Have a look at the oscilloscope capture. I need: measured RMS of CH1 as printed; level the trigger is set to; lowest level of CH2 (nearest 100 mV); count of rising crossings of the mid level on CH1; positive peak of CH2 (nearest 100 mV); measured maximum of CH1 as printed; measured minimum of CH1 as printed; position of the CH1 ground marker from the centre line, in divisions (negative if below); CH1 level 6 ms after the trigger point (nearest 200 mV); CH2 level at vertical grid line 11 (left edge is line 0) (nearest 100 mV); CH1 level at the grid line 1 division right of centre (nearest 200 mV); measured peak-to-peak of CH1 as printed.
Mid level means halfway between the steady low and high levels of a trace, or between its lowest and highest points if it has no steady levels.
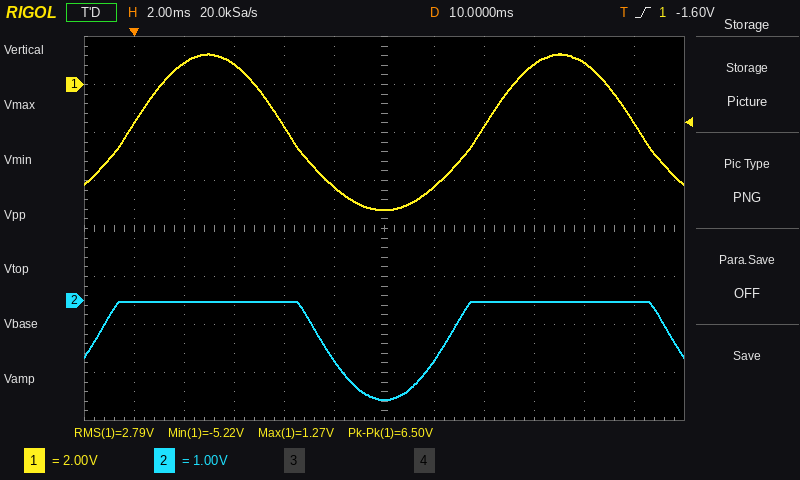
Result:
2.79 V
-1.60 V
-2.1 V
2
0.0 V
1.27 V
-5.22 V
+3.0 div
-1.8 V
0.0 V
-4.2 V
6.50 V
